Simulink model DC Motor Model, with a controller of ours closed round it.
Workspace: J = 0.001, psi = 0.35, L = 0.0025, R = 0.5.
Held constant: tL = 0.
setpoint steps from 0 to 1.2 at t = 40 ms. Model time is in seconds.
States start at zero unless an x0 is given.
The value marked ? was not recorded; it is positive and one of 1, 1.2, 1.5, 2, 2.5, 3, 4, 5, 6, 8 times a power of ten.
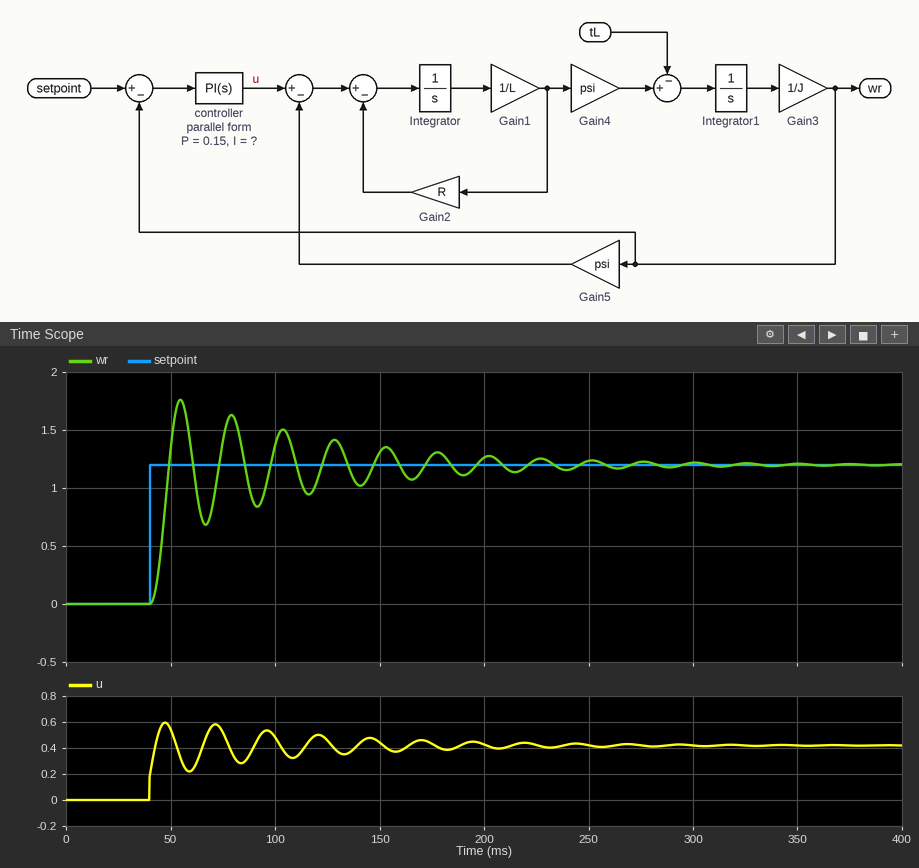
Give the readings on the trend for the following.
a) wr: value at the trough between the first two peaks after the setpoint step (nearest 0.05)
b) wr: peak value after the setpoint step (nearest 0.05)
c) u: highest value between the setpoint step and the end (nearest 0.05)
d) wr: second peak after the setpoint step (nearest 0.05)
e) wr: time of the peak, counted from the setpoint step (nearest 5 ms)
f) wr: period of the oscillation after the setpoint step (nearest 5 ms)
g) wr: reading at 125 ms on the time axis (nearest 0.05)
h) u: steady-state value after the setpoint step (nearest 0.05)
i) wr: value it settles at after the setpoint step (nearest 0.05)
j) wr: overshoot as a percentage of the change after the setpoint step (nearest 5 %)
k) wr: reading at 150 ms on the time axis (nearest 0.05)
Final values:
0.70
1.75
0.60
1.65
15 ms
25 ms
1.35
0.40
1.20
45 %
1.30
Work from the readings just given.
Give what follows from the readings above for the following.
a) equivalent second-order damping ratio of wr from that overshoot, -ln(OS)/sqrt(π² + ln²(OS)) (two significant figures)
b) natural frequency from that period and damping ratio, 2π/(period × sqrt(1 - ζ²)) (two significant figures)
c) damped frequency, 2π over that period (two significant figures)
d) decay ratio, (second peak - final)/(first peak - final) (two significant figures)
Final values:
0.25
0.26 rad/ms
0.25 rad/ms
0.82
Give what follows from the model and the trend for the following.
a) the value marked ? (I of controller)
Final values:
80
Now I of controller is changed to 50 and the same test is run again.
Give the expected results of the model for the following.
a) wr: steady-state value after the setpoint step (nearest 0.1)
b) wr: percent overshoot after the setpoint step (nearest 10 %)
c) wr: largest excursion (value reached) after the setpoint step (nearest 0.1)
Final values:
1.2
20 %
1.4
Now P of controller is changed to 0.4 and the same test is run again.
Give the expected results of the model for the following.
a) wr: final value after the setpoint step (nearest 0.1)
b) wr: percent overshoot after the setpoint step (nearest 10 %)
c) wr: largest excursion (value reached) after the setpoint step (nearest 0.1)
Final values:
1.2
30 %
1.6
